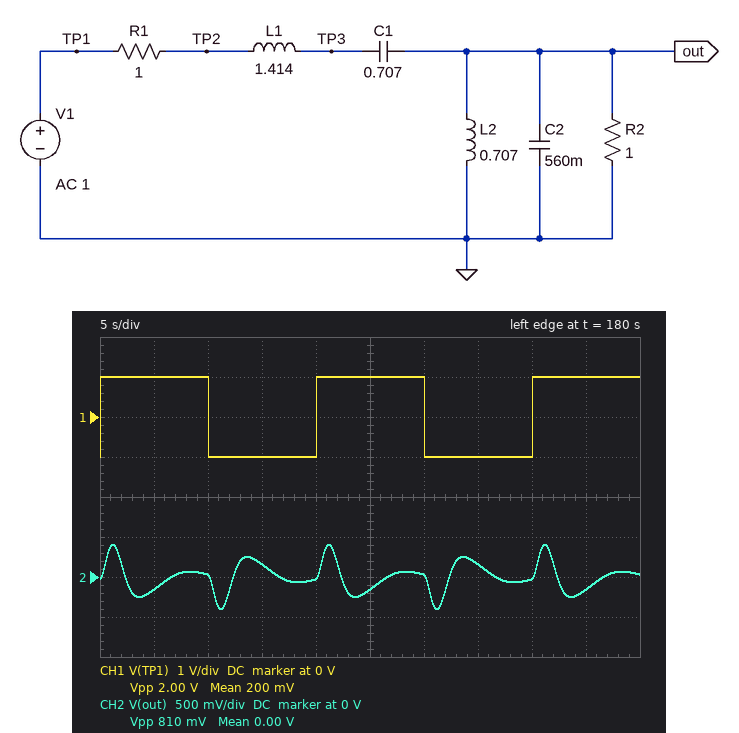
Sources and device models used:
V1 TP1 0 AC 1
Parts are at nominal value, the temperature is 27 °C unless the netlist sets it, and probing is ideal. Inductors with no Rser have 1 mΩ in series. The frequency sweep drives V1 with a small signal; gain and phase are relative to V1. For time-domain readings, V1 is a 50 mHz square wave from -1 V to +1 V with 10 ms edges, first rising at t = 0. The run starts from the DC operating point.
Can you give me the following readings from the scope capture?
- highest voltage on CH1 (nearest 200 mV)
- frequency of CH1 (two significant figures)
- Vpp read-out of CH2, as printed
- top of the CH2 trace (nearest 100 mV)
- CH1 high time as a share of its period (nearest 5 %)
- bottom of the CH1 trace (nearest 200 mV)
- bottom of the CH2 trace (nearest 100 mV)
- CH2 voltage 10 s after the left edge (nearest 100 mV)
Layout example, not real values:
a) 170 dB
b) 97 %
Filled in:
a) 1.0 V
b) 50 mHz
c) 810 mV
d) 400 mV
e) 50 %
f) -1.0 V
g) -400 mV
h) 0 V
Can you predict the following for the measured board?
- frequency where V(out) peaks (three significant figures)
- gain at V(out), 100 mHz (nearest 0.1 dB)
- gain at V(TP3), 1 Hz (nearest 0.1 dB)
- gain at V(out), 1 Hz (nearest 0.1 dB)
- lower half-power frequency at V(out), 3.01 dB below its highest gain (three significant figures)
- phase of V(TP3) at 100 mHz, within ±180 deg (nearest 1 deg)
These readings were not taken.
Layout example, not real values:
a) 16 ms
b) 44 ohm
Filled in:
a) 149 mHz
b) -10.4 dB
c) -24.4 dB
d) -29.3 dB
e) 104 mHz
f) -45 deg
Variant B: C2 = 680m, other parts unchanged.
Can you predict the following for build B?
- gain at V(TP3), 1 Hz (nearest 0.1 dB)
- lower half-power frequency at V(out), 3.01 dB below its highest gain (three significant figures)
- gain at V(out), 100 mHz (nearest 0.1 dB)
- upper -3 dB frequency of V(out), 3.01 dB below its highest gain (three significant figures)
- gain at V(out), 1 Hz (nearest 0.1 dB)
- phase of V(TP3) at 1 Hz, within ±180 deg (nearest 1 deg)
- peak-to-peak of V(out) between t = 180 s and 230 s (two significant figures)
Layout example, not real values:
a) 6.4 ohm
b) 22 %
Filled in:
a) -25.3 dB
b) 103 mHz
c) -10.2 dB
d) 330 mHz
e) -31.0 dB
f) -166 deg
g) 790 mV
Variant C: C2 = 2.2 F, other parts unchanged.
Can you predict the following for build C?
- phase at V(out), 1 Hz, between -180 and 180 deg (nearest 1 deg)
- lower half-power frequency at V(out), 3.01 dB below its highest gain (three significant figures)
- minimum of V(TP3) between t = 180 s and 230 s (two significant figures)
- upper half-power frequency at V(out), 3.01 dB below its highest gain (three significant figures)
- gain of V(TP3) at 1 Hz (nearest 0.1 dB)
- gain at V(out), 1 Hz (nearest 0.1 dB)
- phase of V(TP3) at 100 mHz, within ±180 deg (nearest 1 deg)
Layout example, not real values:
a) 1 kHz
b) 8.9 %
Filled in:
a) -169 deg
b) 90.1 mHz
c) -1.4 V
d) 220 mHz
e) -29.2 dB
f) -41.4 dB
g) -43 deg
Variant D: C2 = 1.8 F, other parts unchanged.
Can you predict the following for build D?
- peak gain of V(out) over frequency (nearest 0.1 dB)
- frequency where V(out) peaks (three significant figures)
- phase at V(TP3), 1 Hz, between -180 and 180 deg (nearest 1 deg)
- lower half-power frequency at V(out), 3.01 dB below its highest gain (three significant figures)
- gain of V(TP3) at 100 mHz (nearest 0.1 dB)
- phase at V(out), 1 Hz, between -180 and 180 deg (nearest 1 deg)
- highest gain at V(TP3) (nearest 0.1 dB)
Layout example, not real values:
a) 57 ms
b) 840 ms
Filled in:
a) -6.2 dB
b) 136 mHz
c) -172 deg
d) 94.4 mHz
e) 0.6 dB
f) -168 deg
g) 1.3 dB
